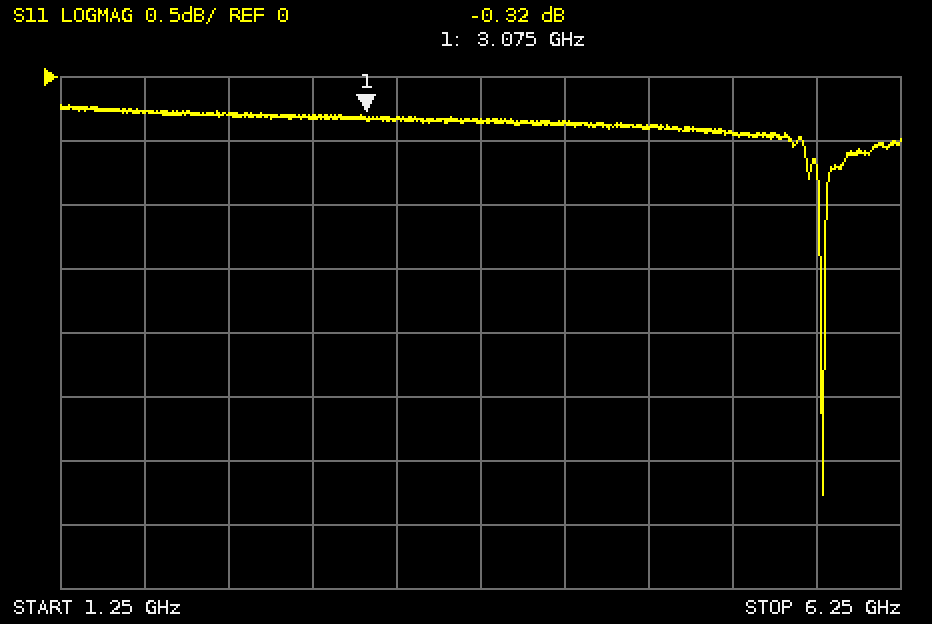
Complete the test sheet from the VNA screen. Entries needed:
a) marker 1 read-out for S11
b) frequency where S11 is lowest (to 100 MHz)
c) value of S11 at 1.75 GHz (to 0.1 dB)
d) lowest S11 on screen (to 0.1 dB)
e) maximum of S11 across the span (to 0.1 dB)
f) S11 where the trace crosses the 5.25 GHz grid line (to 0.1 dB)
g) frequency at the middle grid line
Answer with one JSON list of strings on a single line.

["-0.32 dB", "5.8 GHz", "-0.3 dB", "-3.3 dB", "-0.2 dB", "-0.4 dB", "3.75 GHz"]
